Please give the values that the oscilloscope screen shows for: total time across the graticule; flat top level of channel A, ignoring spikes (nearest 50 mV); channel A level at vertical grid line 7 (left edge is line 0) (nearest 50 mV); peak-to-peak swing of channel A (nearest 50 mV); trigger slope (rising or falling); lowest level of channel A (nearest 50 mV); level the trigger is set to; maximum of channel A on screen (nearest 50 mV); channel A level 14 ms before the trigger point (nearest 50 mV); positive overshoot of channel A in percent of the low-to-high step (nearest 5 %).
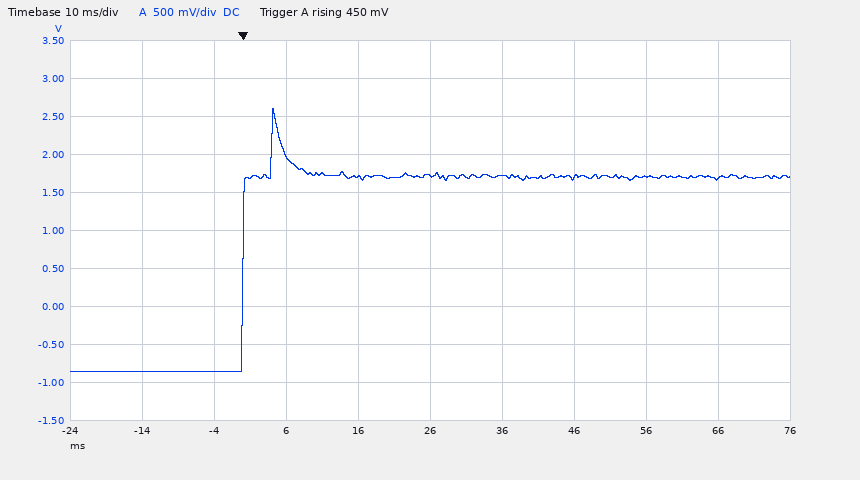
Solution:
100 ms
1.70 V
1.70 V
3.45 V
rising
-850 mV
450 mV
2.60 V
-850 mV
35 %
